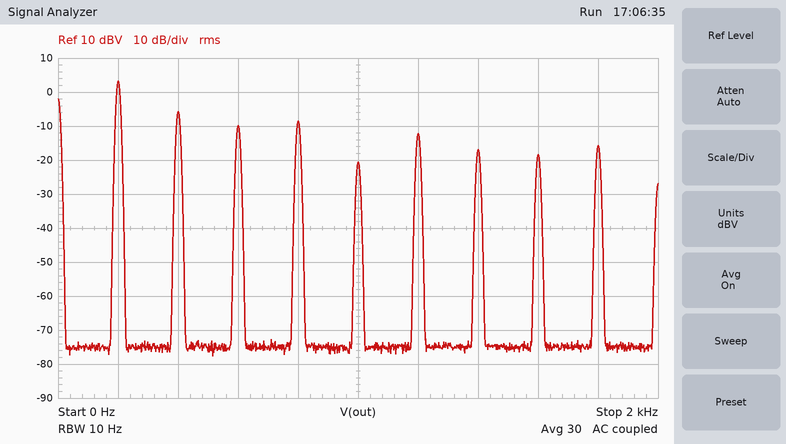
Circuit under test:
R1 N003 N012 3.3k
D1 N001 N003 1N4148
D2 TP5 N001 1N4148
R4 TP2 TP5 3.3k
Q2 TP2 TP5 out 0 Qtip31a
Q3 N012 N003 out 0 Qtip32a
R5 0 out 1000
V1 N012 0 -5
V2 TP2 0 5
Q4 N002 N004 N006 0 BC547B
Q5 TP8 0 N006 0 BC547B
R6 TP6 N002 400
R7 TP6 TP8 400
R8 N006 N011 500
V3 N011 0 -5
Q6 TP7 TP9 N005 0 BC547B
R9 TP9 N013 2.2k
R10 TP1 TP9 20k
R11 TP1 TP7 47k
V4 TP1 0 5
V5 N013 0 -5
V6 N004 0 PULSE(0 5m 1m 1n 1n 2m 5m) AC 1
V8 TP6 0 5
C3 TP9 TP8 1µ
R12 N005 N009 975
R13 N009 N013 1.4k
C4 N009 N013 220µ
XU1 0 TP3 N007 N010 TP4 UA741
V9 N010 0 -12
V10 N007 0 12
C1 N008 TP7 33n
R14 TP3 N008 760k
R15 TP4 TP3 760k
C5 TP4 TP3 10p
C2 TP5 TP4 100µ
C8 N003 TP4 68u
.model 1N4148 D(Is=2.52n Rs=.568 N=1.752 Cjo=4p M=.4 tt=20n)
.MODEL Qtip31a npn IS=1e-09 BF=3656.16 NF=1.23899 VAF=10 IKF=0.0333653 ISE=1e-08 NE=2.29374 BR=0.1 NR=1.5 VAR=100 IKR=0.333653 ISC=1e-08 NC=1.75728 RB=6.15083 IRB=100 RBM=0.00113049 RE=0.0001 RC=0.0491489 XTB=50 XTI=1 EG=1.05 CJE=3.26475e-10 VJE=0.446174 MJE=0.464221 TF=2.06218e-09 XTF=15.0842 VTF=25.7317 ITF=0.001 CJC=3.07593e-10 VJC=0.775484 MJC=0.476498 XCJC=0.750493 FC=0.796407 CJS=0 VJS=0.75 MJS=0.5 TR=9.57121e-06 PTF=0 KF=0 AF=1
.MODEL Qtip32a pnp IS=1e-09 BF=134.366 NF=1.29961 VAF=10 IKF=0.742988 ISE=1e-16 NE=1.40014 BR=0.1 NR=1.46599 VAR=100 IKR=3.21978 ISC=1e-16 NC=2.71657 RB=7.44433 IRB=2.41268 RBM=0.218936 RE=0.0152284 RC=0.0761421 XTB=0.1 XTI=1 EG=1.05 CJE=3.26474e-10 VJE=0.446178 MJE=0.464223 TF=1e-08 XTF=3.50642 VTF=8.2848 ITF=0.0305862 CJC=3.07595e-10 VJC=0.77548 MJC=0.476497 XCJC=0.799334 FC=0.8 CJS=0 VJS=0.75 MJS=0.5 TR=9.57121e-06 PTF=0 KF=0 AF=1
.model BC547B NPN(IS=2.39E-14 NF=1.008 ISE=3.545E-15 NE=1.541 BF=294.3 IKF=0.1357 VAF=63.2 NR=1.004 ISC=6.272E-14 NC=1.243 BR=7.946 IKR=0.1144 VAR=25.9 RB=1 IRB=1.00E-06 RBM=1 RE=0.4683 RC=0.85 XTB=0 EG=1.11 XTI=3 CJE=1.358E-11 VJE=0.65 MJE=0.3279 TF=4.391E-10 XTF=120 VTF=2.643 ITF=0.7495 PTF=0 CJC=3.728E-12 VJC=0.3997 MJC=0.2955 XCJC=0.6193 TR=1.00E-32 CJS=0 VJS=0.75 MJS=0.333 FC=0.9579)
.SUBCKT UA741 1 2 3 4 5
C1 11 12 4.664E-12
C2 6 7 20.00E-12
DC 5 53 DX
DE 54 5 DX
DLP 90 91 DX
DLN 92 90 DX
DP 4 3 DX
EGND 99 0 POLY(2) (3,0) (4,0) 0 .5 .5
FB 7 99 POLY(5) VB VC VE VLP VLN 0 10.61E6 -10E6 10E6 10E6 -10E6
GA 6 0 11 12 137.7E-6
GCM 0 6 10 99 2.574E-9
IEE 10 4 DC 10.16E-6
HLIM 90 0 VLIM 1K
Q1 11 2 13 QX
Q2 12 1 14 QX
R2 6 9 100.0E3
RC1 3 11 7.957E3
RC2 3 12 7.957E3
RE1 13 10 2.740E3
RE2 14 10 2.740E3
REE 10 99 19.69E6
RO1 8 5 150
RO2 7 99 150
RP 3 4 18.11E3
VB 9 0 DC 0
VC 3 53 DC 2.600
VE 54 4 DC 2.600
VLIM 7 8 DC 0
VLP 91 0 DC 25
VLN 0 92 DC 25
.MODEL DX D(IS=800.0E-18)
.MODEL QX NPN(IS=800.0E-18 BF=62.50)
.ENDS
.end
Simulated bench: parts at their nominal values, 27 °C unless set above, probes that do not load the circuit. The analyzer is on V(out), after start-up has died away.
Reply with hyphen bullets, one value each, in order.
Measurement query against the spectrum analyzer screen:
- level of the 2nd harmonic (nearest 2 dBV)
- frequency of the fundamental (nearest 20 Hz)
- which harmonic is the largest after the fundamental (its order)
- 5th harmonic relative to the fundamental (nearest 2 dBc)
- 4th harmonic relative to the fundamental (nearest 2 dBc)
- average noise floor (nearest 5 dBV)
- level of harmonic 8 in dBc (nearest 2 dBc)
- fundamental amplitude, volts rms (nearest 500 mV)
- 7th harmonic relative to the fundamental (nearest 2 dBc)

- -6 dBV
- 200 Hz
- 2
- -24 dBc
- -12 dBc
- -75 dBV
- -22 dBc
- 1.5 V
- -20 dBc
